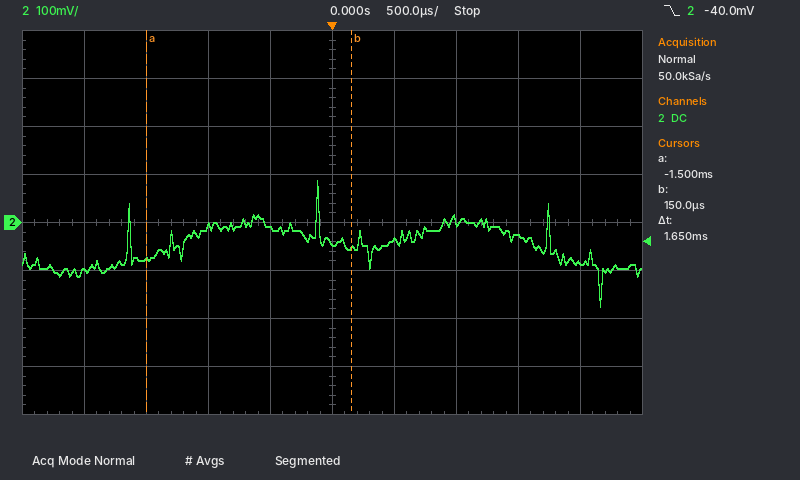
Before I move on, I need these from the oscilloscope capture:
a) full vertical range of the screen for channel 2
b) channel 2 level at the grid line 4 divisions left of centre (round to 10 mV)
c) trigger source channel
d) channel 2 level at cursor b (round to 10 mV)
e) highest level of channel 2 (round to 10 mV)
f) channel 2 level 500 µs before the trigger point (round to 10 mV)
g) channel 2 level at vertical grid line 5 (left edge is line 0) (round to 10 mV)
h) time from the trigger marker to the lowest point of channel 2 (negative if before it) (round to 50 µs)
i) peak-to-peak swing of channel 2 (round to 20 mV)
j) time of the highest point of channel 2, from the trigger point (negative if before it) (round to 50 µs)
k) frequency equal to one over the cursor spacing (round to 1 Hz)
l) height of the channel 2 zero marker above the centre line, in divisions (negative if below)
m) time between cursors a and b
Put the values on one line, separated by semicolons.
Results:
800 mV; -100 mV; channel 2; -50 mV; 90 mV; -10 mV; -40 mV; +2.15 ms; 260 mV; -100 µs; 606 Hz; 0.0 div; 1.65 ms
